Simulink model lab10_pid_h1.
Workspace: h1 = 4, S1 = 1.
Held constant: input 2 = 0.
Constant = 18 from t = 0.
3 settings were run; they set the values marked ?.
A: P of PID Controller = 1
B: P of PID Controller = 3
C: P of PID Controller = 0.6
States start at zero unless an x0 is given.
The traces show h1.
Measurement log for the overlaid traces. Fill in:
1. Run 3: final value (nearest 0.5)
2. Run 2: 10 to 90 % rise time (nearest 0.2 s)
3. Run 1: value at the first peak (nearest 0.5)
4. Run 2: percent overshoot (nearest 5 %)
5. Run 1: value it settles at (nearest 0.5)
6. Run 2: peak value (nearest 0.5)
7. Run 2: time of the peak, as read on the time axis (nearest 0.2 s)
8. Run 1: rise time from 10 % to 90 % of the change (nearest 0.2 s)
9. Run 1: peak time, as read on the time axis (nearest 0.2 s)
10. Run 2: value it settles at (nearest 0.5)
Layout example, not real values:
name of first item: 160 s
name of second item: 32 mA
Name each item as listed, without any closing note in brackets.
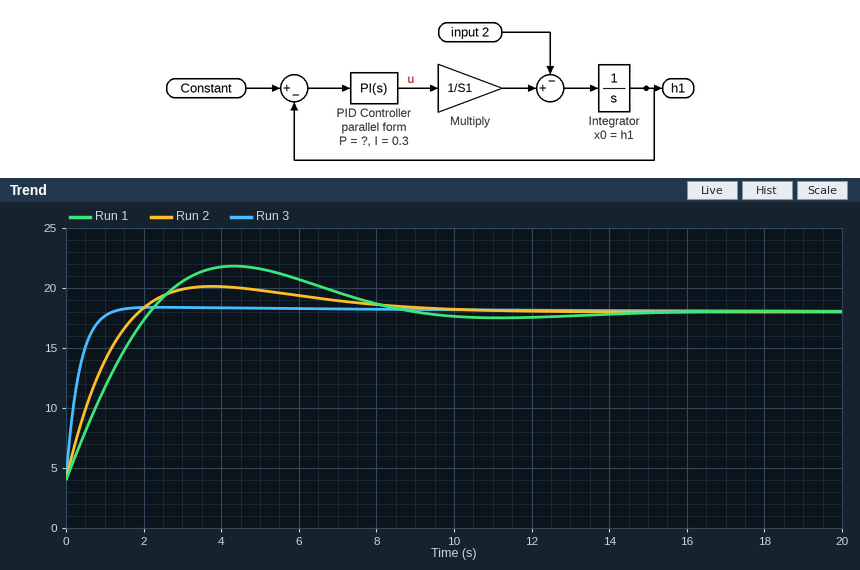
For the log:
Run 3: final value: 18.0
Run 2: 10 to 90 % rise time: 1.4 s
Run 1: value at the first peak: 22.0
Run 2: percent overshoot: 15 %
Run 1: value it settles at: 18.0
Run 2: peak value: 20.0
Run 2: time of the peak, as read on the time axis: 3.8 s
Run 1: rise time from 10 % to 90 % of the change: 1.6 s
Run 1: peak time, as read on the time axis: 4.4 s
Run 2: value it settles at: 18.0
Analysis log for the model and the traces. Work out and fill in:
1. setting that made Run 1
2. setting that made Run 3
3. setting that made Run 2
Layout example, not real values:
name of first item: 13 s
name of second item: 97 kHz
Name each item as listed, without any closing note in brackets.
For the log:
setting that made Run 1: C
setting that made Run 3: B
setting that made Run 2: A
